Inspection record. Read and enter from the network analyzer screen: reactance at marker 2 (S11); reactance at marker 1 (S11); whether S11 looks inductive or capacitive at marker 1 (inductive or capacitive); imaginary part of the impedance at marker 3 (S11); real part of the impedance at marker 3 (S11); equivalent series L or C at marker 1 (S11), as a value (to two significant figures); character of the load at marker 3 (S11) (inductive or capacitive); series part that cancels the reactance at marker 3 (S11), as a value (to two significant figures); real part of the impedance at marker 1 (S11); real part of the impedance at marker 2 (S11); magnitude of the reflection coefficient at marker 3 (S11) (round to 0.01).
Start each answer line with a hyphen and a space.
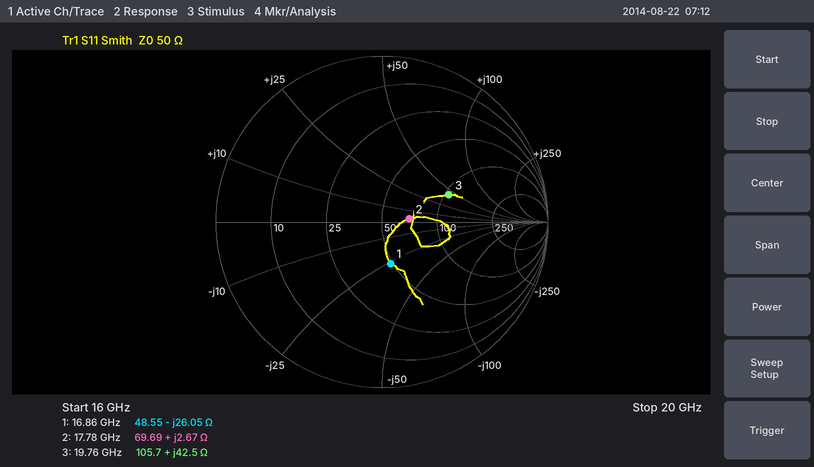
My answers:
- +2.67 Ω
- -26.05 Ω
- capacitive
- +42.5 Ω
- 105.7 Ω
- 360 fF
- inductive
- 190 fF
- 48.55 Ω
- 69.69 Ω
- 0.43
